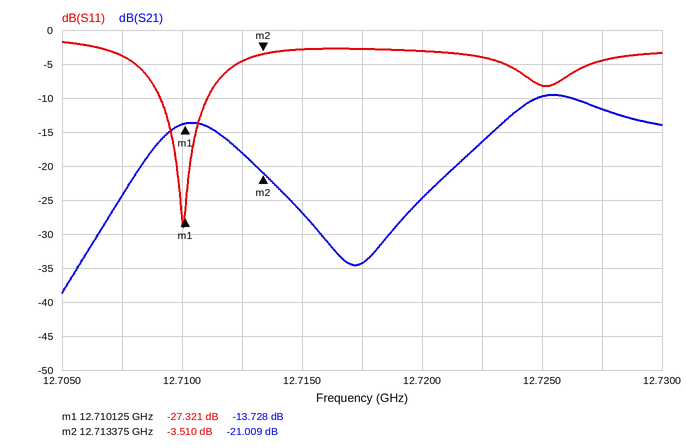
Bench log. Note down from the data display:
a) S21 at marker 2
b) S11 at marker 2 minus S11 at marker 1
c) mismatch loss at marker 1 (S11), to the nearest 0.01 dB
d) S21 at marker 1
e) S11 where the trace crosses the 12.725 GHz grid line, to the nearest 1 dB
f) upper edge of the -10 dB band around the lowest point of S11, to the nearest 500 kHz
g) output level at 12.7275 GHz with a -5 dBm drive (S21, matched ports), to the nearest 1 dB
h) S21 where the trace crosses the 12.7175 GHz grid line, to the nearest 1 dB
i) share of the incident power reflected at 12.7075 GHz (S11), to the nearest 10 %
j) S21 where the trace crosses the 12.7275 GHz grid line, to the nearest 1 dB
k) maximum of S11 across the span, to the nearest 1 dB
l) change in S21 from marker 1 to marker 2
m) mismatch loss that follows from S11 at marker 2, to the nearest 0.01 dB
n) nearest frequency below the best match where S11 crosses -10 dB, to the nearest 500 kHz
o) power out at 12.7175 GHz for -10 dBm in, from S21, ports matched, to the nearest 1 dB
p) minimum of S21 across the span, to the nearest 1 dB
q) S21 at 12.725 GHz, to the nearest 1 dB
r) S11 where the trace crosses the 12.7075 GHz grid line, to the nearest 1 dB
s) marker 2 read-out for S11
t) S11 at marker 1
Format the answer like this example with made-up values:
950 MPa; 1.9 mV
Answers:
-21.009 dB; 23.811 dB; 0.01 dB; -13.728 dB; -8 dB; 12.7110 GHz; -17 dBm; -34 dB; 40 %; -12 dB; -2 dB; -7.281 dB; 2.56 dB; 12.7090 GHz; -44 dBm; -39 dB; -10 dB; -4 dB; -3.510 dB; -27.321 dB
